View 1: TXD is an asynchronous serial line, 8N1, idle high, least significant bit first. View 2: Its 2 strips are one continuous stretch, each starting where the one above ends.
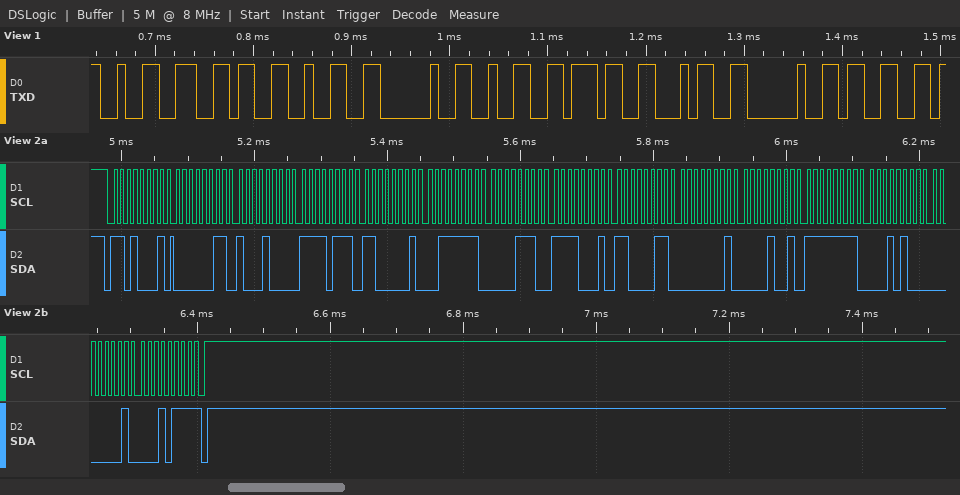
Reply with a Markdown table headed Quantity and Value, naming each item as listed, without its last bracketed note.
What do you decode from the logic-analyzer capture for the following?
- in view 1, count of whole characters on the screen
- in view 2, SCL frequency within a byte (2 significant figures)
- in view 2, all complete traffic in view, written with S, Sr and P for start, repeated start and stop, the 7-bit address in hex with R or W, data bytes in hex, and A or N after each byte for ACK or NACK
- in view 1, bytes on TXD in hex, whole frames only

| Quantity | Value |
|---|---|
| in view 1, count of whole characters on the screen | 9 |
| in view 2, SCL frequency within a byte | 100 kHz |
| in view 2, all complete traffic in view, written with S, Sr and P for start, repeated start and stop, the 7-bit address in hex with R or W, data bytes in hex, and A or N after each byte for ACK or NACK | S 68R A 03 A 88 A F7 A C1 A 3F A 0E A F1 A C3 A 01 A 09 A FF A 14 A 01 A 17 N P |
| in view 1, bytes on TXD in hex, whole frames only | 32 36 32 20 32 37 34 20 33 |
